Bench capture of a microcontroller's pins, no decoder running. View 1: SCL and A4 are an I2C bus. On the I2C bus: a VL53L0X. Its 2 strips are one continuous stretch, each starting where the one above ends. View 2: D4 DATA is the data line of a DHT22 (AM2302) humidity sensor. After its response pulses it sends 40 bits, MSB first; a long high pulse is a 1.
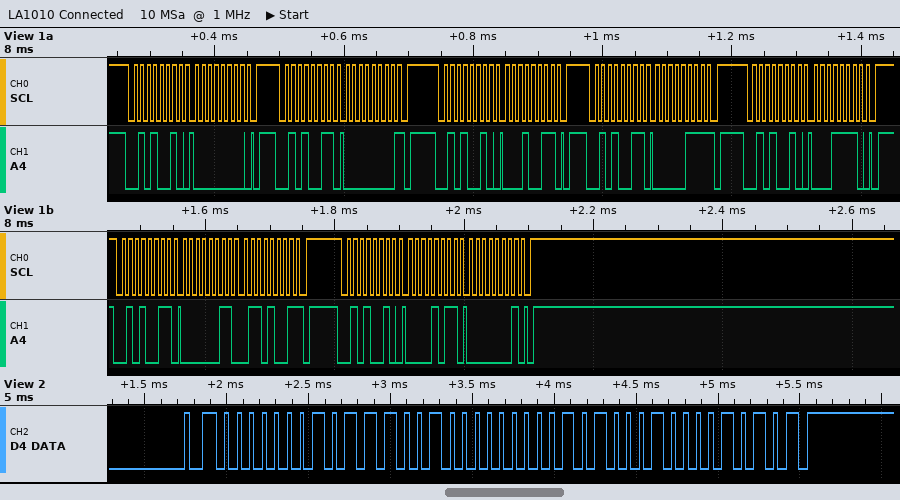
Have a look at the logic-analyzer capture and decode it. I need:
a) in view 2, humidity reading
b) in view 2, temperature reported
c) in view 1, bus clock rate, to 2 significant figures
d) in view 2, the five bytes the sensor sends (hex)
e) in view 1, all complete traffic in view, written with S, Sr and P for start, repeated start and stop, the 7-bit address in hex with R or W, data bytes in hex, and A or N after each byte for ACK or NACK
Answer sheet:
37.0 %
16.2 °C
100 kHz
01 72 00 A2 15
S 29W A 00 A P S 29R A 00 N P S 29W A 13 A P S 29R A 07 N P S 29W A 1E A P S 29R A 03 A 69 N P S 29W A 0B A 01 A P
